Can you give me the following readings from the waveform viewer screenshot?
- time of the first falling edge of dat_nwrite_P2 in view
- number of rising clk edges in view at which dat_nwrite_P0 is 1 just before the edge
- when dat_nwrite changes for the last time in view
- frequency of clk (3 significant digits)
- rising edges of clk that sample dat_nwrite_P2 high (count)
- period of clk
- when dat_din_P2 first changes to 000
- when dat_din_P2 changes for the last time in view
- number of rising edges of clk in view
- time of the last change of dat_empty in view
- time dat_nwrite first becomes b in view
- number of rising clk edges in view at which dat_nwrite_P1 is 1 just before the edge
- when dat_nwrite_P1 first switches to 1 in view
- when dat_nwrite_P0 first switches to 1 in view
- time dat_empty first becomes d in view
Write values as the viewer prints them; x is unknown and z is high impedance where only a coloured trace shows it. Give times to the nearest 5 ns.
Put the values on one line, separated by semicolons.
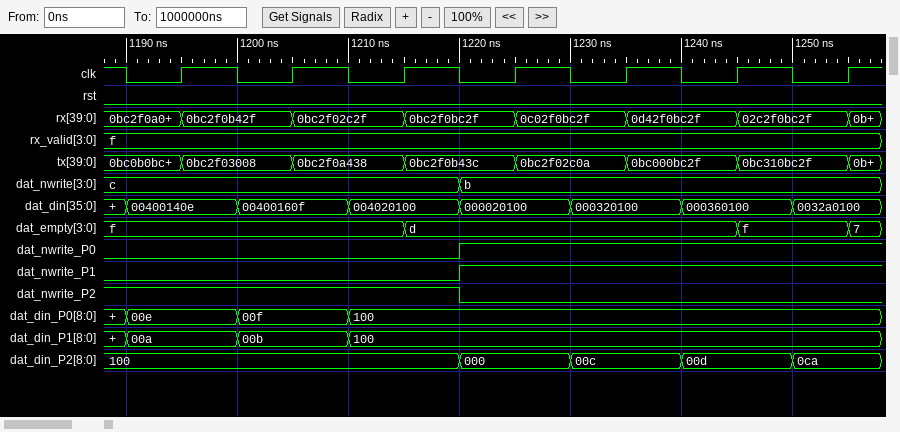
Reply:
1220 ns; 4; 1220 ns; 100 MHz; 3; 10 ns; 1220 ns; 1250 ns; 7; 1255 ns; 1220 ns; 4; 1220 ns; 1220 ns; 1215 ns
